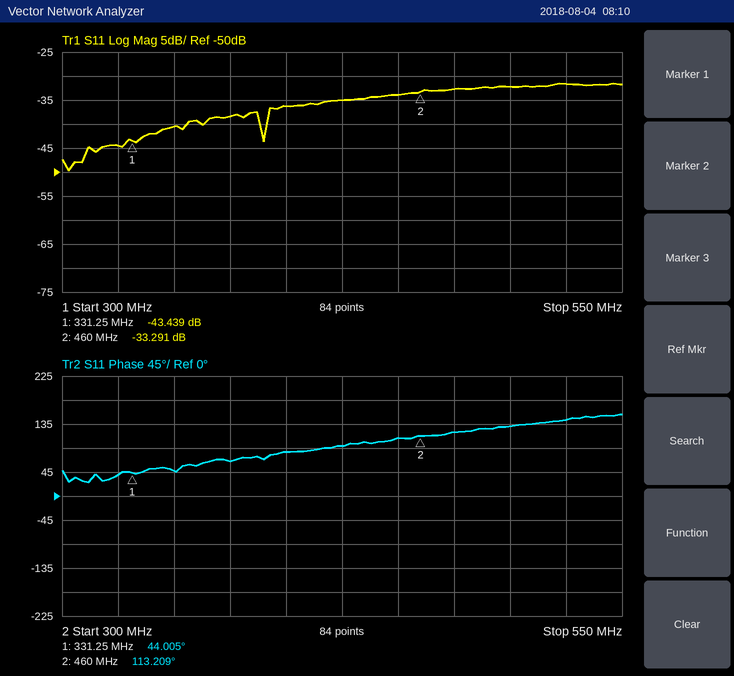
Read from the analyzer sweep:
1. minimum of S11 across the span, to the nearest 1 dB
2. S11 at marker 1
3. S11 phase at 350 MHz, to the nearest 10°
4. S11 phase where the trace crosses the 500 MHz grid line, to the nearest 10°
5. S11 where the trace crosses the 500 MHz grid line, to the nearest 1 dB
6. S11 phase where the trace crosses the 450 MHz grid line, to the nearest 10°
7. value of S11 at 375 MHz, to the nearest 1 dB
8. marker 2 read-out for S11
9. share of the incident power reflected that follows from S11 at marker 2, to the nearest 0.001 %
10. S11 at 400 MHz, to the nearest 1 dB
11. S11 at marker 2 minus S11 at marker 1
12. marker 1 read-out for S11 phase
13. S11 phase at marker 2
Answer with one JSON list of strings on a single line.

["-50 dB", "-43.439 dB", "50°", "130°", "-32 dB", "110°", "-38 dB", "-33.291 dB", "0.047 %", "-36 dB", "10.148 dB", "44.005°", "113.209°"]
